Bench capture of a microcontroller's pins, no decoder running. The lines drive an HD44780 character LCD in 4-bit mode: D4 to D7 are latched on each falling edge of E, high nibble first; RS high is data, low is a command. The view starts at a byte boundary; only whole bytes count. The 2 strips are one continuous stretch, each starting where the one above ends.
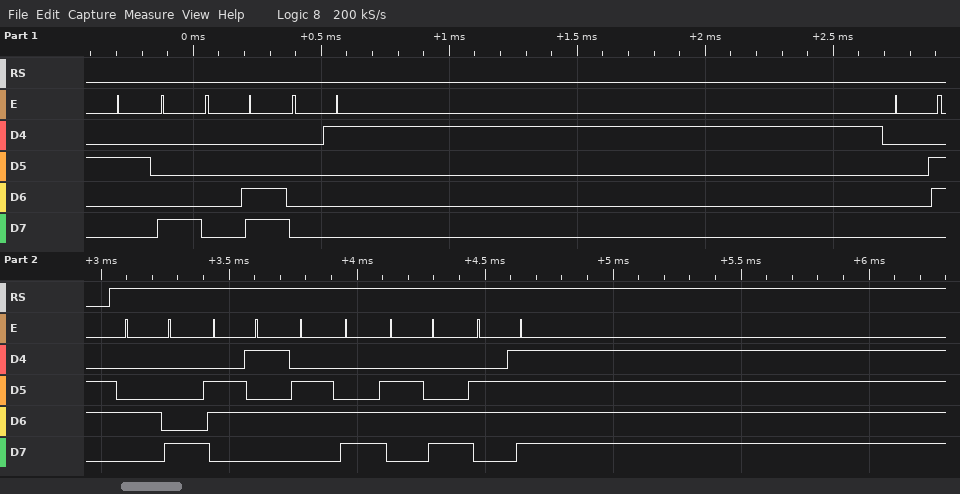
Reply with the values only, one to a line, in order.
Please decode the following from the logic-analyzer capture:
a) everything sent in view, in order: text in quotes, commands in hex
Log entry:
0x28 0x0C 0x01 0x06 "Hello"
